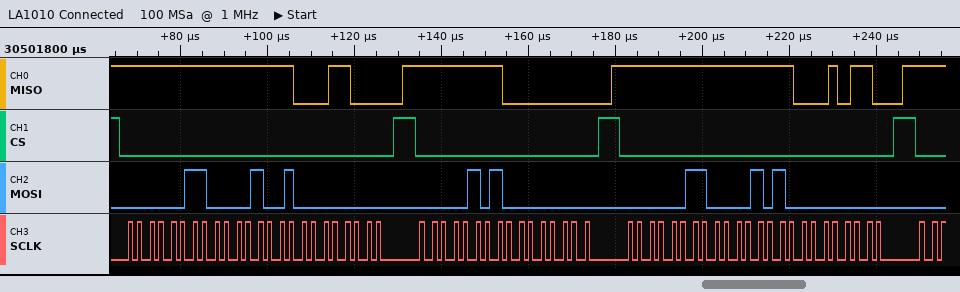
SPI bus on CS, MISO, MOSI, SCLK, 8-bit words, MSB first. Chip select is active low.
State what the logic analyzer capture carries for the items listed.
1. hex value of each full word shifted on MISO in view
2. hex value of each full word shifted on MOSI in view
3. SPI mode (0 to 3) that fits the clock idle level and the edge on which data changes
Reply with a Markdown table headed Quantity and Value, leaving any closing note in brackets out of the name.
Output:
| Quantity | Value |
|---|---|
| hex value of each full word shifted on MISO in view | FF, FF, 18, FF, 00, FF, FF, 16 |
| hex value of each full word shifted on MOSI in view | 03, 09, 00, 05, 00, 03, 0A, 00 |
| SPI mode (0 to 3) that fits the clock idle level and the edge on which data changes | 0 |
